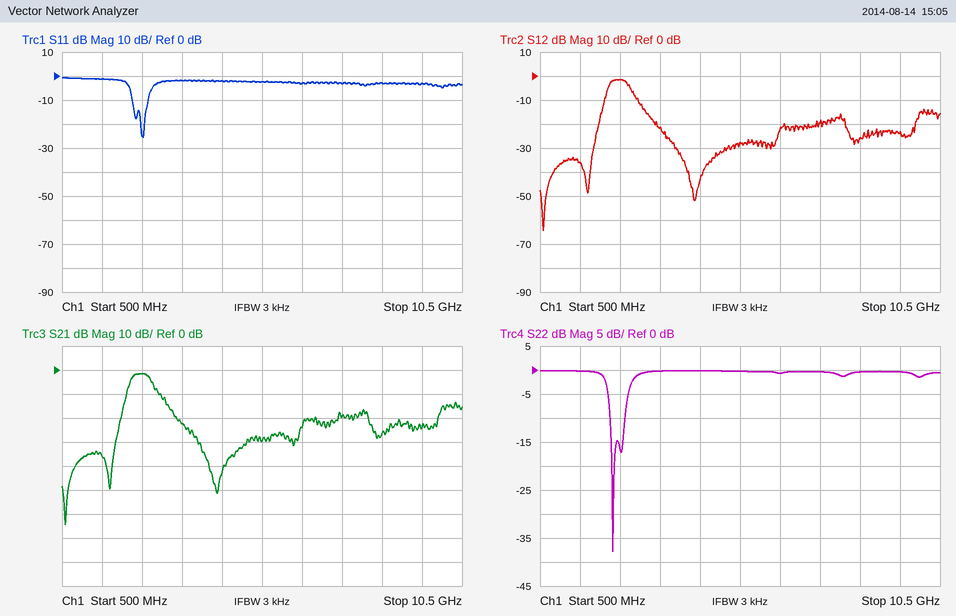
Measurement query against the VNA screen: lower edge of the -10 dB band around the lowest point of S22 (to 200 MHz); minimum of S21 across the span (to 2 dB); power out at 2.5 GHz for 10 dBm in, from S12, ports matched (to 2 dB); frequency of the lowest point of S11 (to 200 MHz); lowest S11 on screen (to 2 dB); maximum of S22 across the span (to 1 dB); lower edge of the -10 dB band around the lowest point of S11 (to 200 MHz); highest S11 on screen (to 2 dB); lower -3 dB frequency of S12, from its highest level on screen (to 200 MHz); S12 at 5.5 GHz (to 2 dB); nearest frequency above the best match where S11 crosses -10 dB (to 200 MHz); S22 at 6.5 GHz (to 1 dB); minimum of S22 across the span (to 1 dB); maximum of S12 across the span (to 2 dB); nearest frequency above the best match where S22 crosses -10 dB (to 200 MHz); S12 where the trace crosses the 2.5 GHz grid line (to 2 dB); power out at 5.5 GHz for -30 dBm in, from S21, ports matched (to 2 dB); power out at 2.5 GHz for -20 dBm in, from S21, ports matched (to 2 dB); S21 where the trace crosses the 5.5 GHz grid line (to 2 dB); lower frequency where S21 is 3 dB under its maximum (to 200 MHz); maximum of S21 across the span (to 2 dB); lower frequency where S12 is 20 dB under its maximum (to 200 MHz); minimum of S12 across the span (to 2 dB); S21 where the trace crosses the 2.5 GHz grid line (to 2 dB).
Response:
2.2 GHz
-64 dB
8 dBm
2.6 GHz
-26 dB
0 dB
2.2 GHz
0 dB
2.2 GHz
-28 dB
2.6 GHz
-1 dB
-38 dB
-2 dB
2.6 GHz
-2 dB
-60 dBm
-22 dBm
-30 dB
2.2 GHz
-2 dB
2.0 GHz
-64 dB
-2 dB
